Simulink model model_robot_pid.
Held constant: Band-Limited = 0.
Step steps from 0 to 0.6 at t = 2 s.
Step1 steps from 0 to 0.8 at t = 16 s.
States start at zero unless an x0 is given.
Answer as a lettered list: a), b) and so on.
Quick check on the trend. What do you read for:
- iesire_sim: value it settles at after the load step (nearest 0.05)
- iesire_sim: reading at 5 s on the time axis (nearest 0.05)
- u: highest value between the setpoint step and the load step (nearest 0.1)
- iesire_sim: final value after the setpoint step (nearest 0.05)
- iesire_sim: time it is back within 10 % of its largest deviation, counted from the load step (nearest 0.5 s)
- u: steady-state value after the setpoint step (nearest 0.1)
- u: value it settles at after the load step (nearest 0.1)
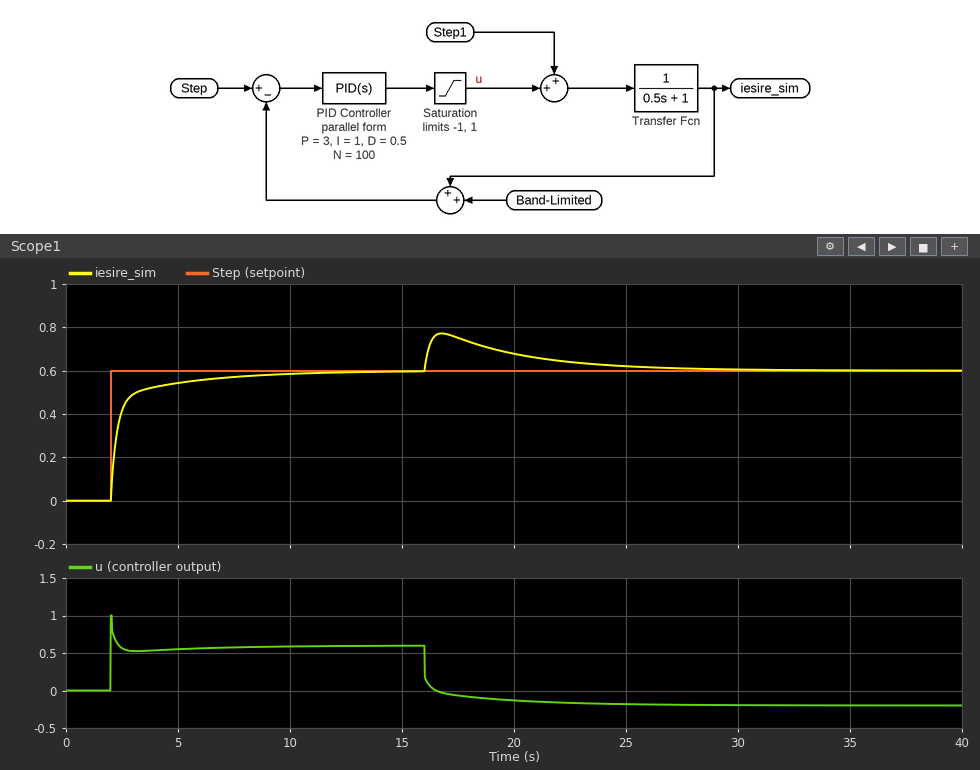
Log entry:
a) 0.60
b) 0.55
c) 1.0
d) 0.60
e) 9.5 s
f) 0.6
g) -0.2
